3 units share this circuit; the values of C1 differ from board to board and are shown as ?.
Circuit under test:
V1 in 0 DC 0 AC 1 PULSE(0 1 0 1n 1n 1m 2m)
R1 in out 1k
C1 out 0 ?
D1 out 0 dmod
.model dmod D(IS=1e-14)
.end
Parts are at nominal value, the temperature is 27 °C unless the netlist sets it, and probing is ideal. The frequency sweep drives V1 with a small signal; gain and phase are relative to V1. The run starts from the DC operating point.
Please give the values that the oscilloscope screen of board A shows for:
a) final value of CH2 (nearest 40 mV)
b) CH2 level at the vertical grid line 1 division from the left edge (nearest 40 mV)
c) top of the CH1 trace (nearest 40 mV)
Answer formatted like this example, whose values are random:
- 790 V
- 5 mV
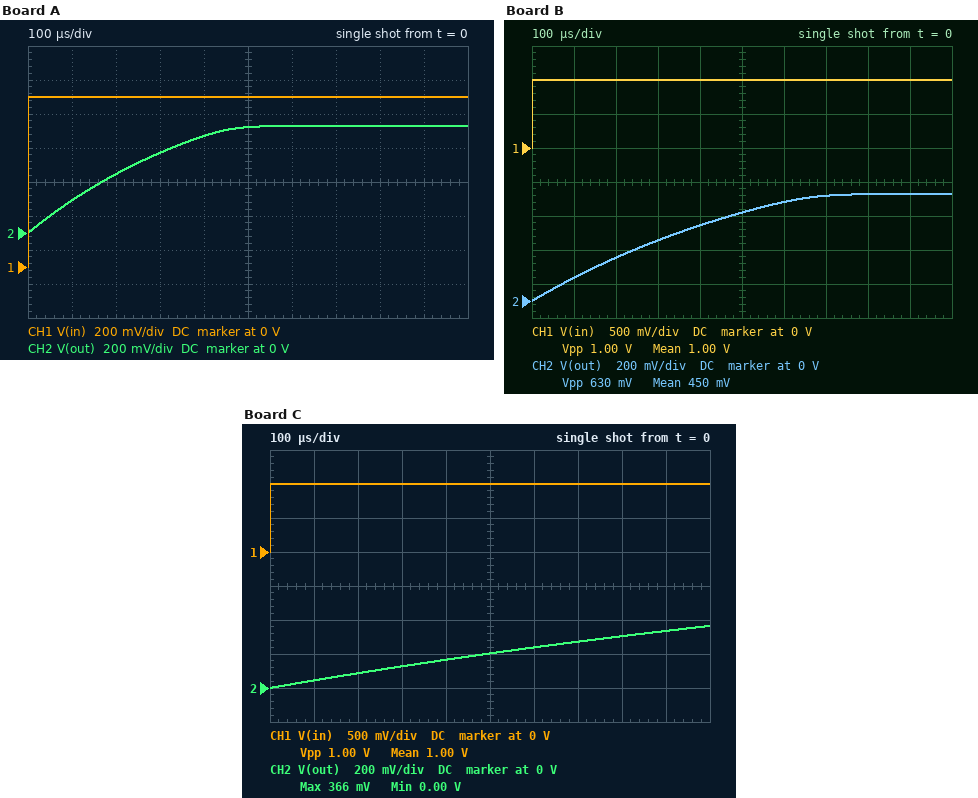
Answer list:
- 640 mV
- 200 mV
- 1.00 V
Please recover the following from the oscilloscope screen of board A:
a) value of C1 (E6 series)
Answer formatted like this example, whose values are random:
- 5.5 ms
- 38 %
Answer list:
- 470 nF
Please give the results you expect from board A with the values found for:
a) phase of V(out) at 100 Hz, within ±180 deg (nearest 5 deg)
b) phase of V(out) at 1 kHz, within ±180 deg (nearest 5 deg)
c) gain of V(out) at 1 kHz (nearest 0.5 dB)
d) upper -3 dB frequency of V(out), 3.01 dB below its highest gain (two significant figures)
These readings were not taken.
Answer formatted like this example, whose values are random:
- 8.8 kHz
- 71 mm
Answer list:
- -15 deg
- -70 deg
- -10.0 dB
- 340 Hz
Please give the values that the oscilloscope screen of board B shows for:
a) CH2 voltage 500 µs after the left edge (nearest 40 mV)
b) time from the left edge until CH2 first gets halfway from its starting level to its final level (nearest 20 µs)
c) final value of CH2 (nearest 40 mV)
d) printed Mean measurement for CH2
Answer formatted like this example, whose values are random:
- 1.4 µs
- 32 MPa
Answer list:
- 520 mV
- 260 µs
- 640 mV
- 450 mV
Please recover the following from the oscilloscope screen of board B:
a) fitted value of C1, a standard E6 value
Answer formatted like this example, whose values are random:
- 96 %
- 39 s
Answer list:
- 680 nF
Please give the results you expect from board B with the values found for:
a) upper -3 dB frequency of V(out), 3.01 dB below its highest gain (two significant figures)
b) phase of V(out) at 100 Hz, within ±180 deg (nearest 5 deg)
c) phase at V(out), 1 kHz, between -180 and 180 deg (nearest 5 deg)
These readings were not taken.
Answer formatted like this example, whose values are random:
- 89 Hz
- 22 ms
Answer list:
- 230 Hz
- -25 deg
- -75 deg
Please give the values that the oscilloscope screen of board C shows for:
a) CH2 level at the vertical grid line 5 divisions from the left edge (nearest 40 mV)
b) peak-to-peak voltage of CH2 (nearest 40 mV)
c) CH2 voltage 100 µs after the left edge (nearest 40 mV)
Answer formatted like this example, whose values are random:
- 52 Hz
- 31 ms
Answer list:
- 200 mV
- 360 mV
- 40 mV
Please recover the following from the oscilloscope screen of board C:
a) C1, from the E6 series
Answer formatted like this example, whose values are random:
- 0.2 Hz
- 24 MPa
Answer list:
- 2.2 µF
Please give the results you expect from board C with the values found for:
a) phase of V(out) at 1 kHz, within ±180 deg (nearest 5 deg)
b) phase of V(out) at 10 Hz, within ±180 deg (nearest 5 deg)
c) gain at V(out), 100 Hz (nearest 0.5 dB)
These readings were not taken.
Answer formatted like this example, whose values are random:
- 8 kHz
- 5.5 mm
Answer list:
- -85 deg
- -10 deg
- -4.5 dB
